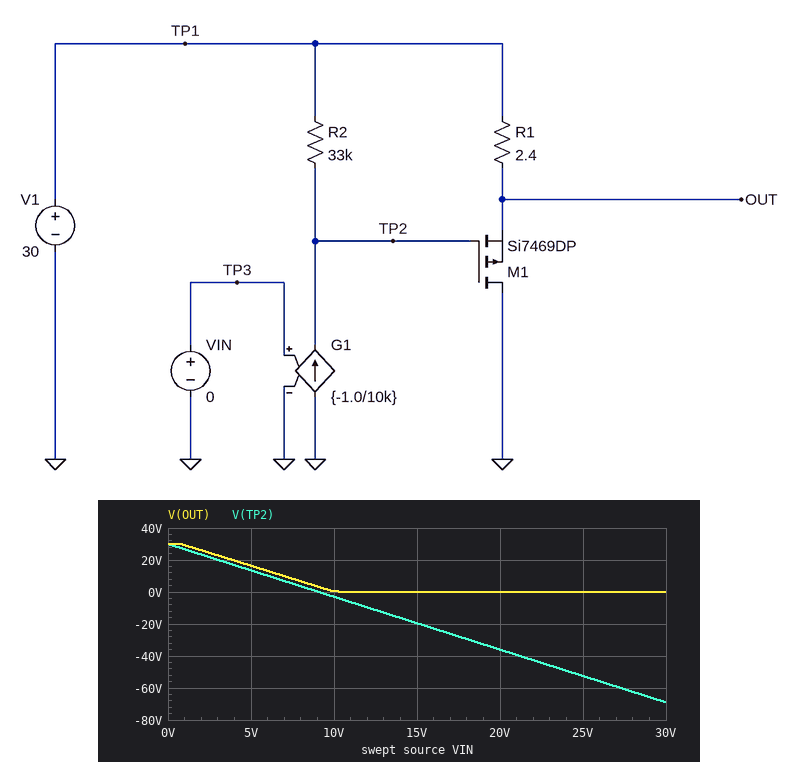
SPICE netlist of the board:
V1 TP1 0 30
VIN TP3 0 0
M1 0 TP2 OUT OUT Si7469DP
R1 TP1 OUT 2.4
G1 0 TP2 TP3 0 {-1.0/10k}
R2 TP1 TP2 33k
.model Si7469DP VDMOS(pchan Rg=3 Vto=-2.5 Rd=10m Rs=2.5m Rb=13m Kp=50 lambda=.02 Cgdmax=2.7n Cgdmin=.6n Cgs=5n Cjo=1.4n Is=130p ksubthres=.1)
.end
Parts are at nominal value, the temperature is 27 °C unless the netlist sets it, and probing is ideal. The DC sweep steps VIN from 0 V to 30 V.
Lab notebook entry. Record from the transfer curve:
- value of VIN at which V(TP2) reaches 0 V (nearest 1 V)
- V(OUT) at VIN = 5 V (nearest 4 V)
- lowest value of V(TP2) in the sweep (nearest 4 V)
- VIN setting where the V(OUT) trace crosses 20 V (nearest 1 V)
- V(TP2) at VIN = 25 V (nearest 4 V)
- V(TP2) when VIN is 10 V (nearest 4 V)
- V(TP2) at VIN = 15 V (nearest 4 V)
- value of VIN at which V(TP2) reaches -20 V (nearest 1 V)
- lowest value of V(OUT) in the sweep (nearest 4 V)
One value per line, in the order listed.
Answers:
9 V
16 V
-68 V
4 V
-52 V
-4 V
-20 V
15 V
0 V
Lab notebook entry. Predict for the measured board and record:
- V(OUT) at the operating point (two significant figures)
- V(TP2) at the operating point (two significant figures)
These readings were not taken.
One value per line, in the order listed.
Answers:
30 V
30 V
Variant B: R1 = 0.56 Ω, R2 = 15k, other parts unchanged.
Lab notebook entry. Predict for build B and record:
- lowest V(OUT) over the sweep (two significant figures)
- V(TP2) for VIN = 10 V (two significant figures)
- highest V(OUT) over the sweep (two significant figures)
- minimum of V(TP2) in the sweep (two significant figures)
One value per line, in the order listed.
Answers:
730 mV
15 V
30 V
-15 V
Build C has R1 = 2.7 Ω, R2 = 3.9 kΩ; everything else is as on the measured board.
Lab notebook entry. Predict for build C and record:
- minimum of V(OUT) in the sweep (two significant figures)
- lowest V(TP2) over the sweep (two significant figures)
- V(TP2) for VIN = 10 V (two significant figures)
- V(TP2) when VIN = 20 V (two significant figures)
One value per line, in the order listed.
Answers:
21 V
18 V
26 V
22 V
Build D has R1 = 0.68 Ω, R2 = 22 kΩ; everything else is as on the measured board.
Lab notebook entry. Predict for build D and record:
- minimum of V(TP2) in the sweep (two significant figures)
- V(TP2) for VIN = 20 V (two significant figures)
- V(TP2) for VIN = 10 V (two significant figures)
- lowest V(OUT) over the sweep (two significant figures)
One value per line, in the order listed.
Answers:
-36 V
-14 V
8.0 V
570 mV
